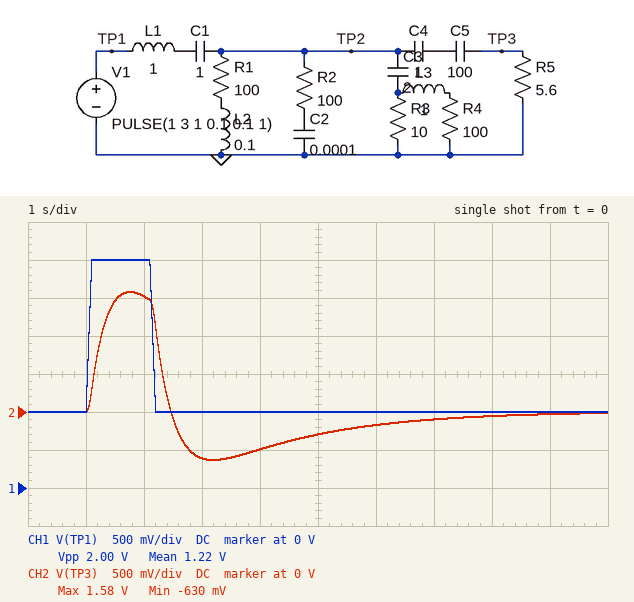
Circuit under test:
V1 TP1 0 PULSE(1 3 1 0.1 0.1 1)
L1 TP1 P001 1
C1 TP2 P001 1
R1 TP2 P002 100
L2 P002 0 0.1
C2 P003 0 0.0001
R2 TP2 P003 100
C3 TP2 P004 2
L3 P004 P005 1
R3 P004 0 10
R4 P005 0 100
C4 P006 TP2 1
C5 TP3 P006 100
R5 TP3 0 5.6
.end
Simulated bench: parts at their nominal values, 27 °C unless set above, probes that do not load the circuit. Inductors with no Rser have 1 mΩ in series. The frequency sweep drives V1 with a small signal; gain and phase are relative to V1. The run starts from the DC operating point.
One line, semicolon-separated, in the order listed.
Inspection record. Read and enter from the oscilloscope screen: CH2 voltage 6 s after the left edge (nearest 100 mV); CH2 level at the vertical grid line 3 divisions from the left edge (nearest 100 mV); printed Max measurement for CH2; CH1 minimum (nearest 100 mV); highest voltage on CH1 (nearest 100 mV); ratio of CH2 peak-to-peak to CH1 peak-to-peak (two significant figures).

-200 mV; -600 mV; 1.58 V; 1.0 V; 3.0 V; 1.1
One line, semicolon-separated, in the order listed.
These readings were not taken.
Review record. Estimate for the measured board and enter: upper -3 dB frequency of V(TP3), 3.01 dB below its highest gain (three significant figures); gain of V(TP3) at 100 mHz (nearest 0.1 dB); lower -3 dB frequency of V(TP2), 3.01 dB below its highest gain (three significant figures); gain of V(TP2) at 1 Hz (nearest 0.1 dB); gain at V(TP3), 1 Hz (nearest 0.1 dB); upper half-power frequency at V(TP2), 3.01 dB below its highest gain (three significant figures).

599 mHz; -1.1 dB; 54.1 mHz; -6.3 dB; -6.3 dB; 589 mHz
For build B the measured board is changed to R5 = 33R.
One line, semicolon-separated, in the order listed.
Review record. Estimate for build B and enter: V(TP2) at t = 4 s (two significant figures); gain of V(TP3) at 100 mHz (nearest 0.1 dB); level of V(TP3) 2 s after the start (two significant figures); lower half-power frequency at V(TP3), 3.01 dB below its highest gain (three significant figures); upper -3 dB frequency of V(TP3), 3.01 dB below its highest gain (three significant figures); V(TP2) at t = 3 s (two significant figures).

-230 mV; -0.2 dB; 1.8 V; 29.3 mHz; 1.09 Hz; -270 mV
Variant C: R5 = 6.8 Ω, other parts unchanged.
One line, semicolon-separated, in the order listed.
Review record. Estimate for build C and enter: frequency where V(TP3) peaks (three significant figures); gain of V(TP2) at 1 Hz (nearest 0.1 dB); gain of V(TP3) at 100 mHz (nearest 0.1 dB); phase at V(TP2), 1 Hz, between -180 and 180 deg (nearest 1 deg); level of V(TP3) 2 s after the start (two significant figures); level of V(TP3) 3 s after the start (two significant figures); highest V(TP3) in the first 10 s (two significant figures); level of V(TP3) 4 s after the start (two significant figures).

191 mHz; -5.6 dB; -0.8 dB; -59 deg; 1.6 V; -570 mV; 1.6 V; -460 mV
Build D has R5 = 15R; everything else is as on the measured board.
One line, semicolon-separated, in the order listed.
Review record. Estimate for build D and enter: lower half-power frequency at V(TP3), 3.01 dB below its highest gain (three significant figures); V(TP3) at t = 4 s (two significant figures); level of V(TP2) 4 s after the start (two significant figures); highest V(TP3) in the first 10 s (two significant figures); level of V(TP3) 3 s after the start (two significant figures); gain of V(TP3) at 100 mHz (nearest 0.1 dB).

37.7 mHz; -350 mV; -260 mV; 1.8 V; -420 mV; -0.3 dB
